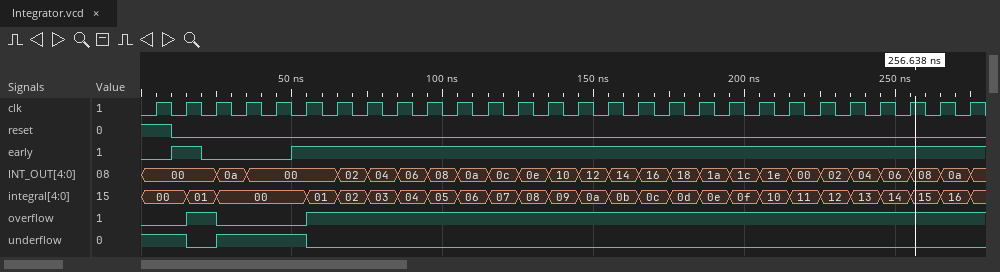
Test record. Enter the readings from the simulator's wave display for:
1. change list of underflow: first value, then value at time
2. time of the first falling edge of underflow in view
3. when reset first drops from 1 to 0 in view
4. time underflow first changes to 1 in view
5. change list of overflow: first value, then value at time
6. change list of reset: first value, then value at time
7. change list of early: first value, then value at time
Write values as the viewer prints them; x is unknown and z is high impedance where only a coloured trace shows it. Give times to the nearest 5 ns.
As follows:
1, 0 at 15 ns, 1 at 25 ns, 0 at 55 ns
15 ns
10 ns
25 ns
0, 1 at 15 ns, 0 at 25 ns, 1 at 55 ns
1, 0 at 10 ns
0, 1 at 10 ns, 0 at 20 ns, 1 at 50 ns
